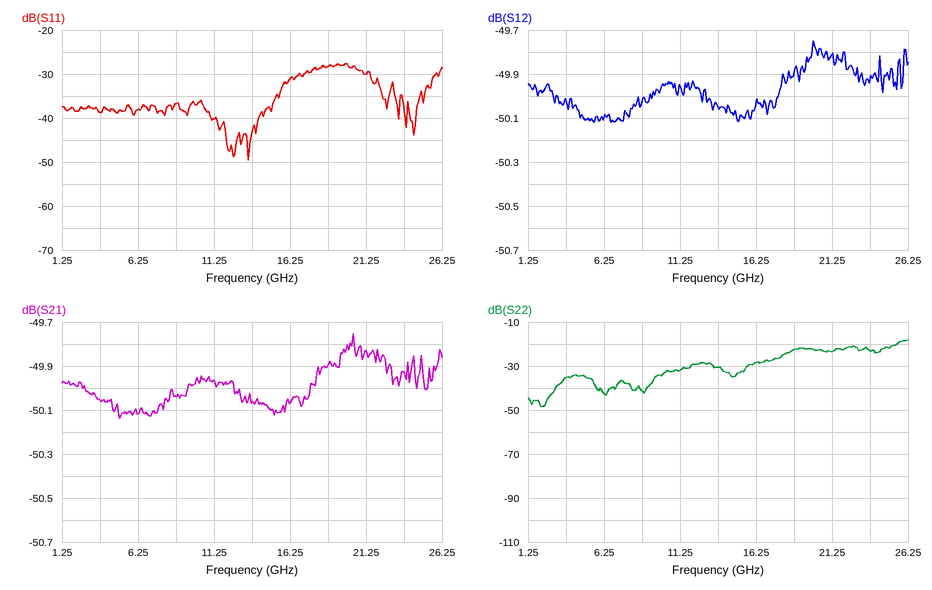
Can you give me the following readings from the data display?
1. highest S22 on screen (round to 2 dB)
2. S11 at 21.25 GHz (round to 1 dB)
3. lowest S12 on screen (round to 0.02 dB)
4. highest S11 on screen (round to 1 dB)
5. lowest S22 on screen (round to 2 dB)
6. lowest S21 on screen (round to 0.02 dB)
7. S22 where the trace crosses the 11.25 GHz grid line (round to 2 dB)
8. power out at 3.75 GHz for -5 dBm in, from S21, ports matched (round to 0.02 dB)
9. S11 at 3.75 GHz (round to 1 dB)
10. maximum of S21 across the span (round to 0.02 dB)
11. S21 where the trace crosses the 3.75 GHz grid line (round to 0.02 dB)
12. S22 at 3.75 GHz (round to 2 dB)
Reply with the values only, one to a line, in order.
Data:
-18 dB
-30 dB
-50.12 dB
-28 dB
-48 dB
-50.14 dB
-32 dB
-55.06 dBm
-39 dB
-49.76 dB
-50.06 dB
-36 dB
